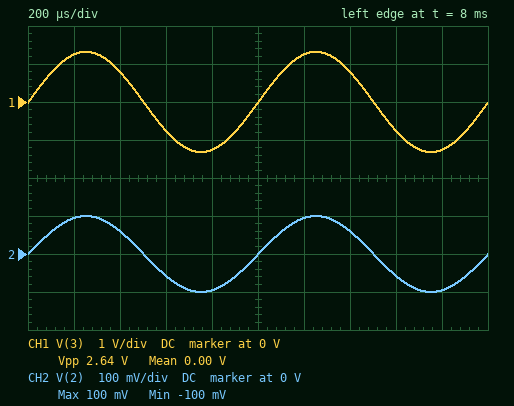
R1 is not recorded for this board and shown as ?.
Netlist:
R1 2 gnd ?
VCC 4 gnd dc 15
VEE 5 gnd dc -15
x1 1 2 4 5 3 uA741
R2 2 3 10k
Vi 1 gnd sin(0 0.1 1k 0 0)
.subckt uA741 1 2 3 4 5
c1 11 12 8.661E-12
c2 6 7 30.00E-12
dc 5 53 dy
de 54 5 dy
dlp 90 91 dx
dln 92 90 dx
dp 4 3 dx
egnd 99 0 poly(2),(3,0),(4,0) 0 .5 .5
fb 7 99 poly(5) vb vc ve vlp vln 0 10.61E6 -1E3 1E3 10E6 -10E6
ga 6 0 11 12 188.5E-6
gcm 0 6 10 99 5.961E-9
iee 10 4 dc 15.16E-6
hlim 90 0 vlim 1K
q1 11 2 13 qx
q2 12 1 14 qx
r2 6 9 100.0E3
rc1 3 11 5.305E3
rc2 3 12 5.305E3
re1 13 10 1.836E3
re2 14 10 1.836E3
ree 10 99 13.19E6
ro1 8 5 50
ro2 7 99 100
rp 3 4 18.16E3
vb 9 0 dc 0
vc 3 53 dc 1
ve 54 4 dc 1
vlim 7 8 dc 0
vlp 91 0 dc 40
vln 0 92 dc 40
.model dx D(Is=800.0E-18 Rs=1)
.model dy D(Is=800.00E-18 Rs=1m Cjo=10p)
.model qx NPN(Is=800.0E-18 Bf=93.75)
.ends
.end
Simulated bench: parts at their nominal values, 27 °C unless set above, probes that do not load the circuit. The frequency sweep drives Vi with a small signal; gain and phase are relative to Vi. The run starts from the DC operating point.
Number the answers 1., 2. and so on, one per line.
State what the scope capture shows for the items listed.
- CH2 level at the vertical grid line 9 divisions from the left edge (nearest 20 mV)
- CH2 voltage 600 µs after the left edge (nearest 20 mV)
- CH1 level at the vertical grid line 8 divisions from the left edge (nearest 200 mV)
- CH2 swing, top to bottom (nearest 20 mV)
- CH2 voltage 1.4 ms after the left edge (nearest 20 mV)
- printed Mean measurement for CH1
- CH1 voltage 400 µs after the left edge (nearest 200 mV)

1. -100 mV
2. -60 mV
3. -800 mV
4. 200 mV
5. 60 mV
6. 0.00 V
7. 800 mV
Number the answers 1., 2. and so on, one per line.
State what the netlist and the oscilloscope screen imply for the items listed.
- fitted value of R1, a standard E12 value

1. 820 Ω
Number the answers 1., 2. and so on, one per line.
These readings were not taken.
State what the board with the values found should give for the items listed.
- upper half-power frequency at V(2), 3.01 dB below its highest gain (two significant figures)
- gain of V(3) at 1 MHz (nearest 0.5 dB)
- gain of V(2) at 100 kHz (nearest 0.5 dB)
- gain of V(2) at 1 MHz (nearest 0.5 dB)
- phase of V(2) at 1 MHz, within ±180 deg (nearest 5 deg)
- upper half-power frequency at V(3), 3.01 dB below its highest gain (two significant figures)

1. 79 kHz
2. -1.0 dB
3. -4.0 dB
4. -23.5 dB
5. -115 deg
6. 79 kHz
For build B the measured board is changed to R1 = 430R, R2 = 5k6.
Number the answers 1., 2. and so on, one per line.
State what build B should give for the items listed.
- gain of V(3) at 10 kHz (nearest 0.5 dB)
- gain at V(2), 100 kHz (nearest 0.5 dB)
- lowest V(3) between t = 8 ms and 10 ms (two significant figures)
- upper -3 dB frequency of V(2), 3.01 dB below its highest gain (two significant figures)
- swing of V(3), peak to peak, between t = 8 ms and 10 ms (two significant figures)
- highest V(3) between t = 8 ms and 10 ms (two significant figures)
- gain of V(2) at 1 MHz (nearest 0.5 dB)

1. 23.0 dB
2. -4.5 dB
3. -1.4 V
4. 74 kHz
5. 2.8 V
6. 1.4 V
7. -24.0 dB
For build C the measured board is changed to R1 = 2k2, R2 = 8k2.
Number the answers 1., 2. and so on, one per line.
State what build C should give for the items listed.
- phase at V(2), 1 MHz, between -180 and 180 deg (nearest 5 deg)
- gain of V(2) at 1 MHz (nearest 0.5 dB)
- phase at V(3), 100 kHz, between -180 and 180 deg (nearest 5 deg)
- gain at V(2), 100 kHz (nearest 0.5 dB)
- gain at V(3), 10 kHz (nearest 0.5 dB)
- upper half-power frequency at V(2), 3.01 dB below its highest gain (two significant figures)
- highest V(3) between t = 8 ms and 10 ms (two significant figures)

1. -110 deg
2. -14.0 dB
3. -25 deg
4. -0.5 dB
5. 13.5 dB
6. 240 kHz
7. 470 mV
